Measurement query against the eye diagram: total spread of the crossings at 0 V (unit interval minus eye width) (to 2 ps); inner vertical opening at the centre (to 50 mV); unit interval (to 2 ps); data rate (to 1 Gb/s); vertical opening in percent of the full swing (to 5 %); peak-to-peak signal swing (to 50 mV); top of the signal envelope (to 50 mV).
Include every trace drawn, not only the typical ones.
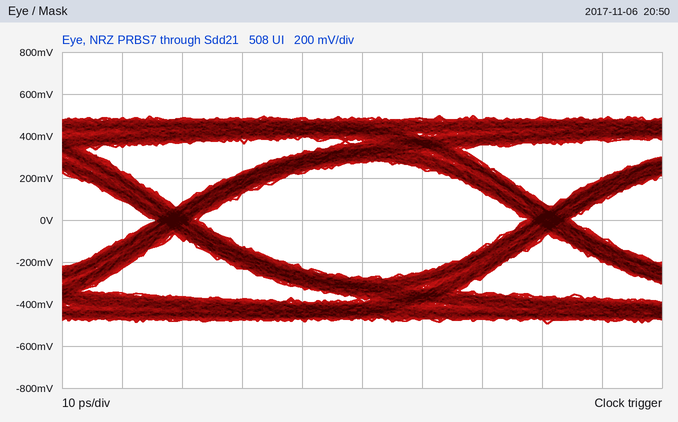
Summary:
8 ps
550 mV
62 ps
16 Gb/s
55 %
1.00 V
500 mV
